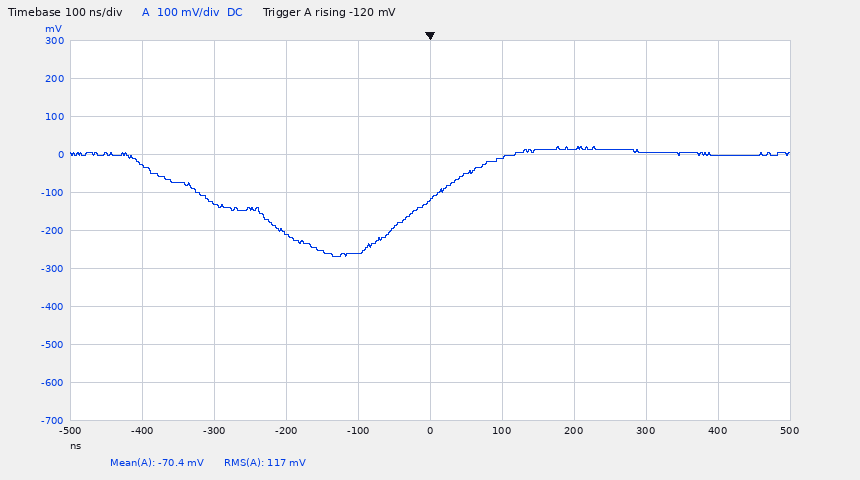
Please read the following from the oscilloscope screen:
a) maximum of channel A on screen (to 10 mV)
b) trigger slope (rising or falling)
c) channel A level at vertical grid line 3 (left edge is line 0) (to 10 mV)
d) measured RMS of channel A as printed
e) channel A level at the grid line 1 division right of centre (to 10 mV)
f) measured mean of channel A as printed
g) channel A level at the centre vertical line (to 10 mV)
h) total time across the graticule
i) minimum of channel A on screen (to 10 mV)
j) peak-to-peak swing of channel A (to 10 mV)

20 mV
rising
-210 mV
117 mV
-10 mV
-70.4 mV
-120 mV
1 µs
-270 mV
290 mV
